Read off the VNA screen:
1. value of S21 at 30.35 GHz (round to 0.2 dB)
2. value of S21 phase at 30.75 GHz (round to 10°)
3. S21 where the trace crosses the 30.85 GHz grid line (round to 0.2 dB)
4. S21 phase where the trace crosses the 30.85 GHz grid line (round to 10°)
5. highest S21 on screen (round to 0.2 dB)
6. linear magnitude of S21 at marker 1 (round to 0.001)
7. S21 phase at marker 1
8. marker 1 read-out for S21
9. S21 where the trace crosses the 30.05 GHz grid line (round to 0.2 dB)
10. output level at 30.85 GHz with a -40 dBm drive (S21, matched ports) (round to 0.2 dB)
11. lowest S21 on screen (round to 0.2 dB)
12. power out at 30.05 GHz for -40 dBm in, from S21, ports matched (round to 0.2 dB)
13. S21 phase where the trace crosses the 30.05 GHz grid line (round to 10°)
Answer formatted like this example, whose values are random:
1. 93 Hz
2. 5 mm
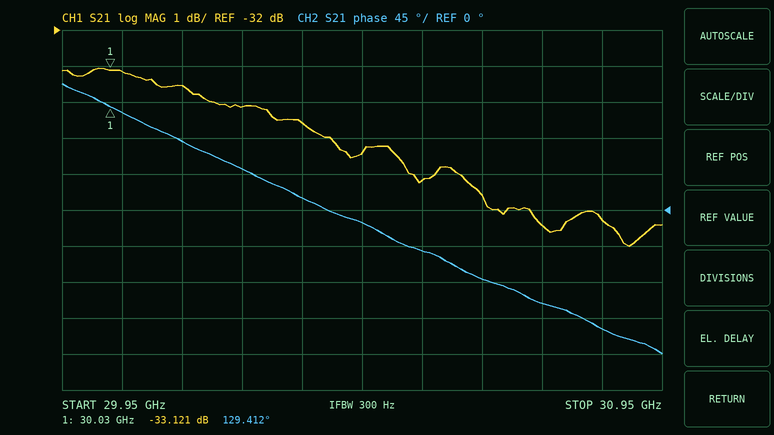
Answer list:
1. -34.6 dB
2. -120°
3. -37.2 dB
4. -150°
5. -33.0 dB
6. 0.022
7. 129.412°
8. -33.121 dB
9. -33.2 dB
10. -77.2 dBm
11. -38.0 dB
12. -73.2 dBm
13. 120°
